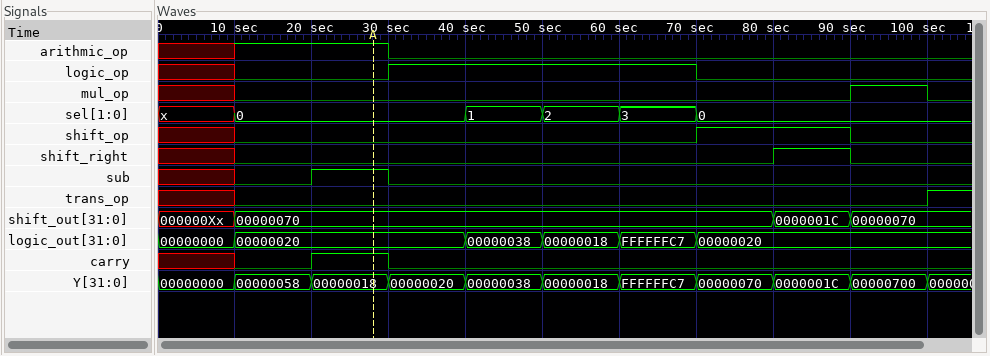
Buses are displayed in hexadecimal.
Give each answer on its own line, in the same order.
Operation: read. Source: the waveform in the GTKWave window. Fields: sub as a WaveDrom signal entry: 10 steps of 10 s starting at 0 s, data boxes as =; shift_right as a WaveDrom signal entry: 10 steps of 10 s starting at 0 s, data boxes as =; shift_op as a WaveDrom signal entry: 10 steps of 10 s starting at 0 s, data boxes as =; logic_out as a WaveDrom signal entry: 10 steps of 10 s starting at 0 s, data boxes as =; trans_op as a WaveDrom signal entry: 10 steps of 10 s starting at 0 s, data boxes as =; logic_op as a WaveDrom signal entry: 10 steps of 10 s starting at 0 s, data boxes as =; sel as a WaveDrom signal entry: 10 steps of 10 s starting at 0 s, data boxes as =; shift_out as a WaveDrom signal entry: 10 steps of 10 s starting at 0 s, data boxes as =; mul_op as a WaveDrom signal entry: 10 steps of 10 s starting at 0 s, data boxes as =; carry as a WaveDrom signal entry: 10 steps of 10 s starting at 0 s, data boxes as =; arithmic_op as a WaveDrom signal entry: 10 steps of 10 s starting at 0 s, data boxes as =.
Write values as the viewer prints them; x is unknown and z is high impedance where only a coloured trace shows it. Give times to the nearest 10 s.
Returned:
{name: 'sub', wave: 'x010......'}
{name: 'shift_right', wave: 'x0......10'}
{name: 'shift_op', wave: 'x0.....1.0'}
{name: 'logic_out', wave: '==..====..', data: '00000000 00000020 00000038 00000018 FFFFFFC7 00000020'}
{name: 'trans_op', wave: 'x0........'}
{name: 'logic_op', wave: 'x0.1...0..'}
{name: 'sel', wave: 'x=..====..', data: '0 1 2 3 0'}
{name: 'shift_out', wave: '==......==', data: '000000Xx 00000070 0000001C 00000070'}
{name: 'mul_op', wave: 'x0.......1'}
{name: 'carry', wave: 'x010......'}
{name: 'arithmic_op', wave: 'x1.0......'}
